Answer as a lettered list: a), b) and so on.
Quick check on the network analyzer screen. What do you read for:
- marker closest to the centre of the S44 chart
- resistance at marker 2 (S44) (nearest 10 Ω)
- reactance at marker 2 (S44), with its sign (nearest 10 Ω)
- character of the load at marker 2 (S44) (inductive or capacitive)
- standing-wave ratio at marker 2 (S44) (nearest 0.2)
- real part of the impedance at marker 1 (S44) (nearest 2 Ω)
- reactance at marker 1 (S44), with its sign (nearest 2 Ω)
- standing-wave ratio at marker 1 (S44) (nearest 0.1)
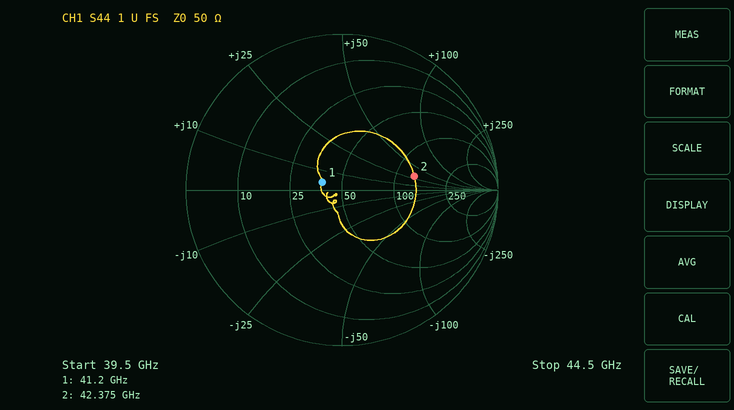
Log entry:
a) marker 1
b) 130 Ω
c) +30 Ω
d) inductive
e) 2.8
f) 38 Ω
g) +4 Ω
h) 1.3
